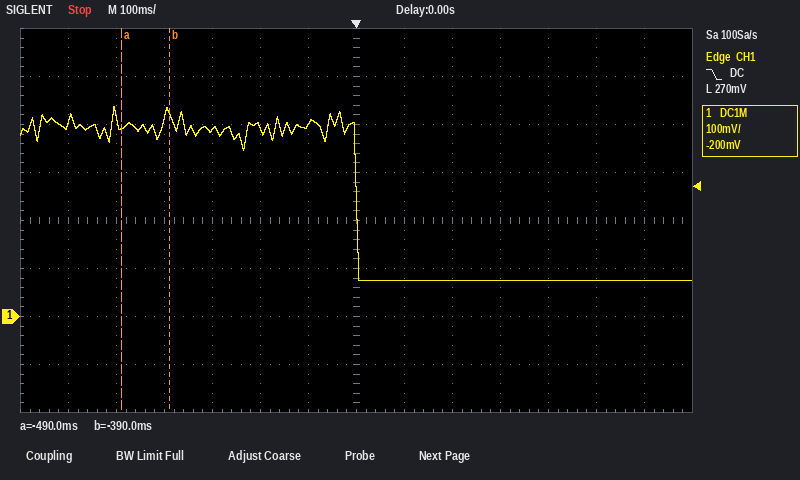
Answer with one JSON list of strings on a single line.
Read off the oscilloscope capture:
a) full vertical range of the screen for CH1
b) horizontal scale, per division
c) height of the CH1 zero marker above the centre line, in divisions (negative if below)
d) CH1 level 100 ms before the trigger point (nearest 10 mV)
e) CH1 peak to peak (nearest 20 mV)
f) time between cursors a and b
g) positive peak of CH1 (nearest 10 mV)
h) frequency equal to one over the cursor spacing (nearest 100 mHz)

["800 mV", "100 ms", "-2.0 div", "400 mV", "360 mV", "100 ms", "440 mV", "10.0 Hz"]
